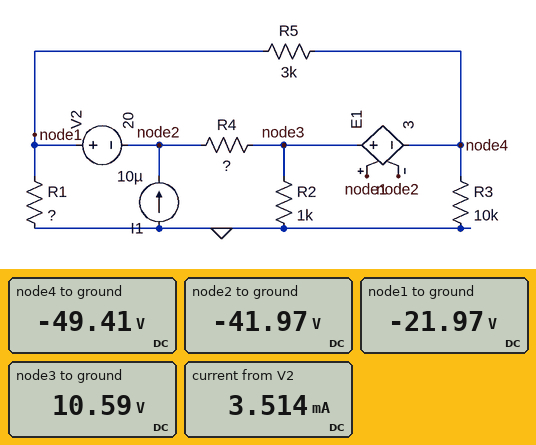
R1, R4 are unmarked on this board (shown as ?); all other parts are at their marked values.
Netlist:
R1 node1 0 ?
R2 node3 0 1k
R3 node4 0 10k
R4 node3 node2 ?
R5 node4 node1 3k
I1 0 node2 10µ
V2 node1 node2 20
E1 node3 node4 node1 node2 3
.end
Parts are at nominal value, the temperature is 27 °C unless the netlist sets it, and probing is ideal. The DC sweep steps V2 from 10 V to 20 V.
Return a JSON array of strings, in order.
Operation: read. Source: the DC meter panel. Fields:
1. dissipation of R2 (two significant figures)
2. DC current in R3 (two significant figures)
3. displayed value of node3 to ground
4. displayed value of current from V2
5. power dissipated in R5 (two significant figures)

["110 mW", "4.9 mA", "10.59 V", "3.514 mA", "250 mW"]
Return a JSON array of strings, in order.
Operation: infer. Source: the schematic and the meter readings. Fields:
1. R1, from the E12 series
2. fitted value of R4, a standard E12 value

["3.9 kΩ", "15 kΩ"]
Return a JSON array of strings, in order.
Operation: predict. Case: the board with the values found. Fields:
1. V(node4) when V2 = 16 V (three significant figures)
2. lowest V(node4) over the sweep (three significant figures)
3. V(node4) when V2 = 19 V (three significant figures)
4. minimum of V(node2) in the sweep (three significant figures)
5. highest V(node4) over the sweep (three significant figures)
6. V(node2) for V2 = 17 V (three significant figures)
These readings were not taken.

["-39.5 V", "-49.4 V", "-46.9 V", "-42.0 V", "-24.7 V", "-35.7 V"]
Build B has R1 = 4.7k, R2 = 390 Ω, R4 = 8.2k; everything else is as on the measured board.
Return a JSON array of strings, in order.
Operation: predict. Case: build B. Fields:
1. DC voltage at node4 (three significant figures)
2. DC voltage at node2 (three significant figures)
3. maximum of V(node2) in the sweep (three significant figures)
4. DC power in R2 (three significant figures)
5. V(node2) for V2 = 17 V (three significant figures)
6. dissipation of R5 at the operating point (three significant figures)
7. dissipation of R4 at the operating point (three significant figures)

["-55.9 V", "-43.5 V", "-21.7 V", "43.7 mW", "-36.9 V", "350 mW", "276 mW"]
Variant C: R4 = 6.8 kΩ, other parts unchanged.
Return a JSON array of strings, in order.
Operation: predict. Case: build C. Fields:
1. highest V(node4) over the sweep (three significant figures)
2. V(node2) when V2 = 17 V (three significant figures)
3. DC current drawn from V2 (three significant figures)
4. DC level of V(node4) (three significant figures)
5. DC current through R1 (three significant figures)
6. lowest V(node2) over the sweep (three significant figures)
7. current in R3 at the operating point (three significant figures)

["-25.3 V", "-31.4 V", "6.84 mA", "-50.6 V", "4.36 mA", "-37.0 V", "5.06 mA"]
